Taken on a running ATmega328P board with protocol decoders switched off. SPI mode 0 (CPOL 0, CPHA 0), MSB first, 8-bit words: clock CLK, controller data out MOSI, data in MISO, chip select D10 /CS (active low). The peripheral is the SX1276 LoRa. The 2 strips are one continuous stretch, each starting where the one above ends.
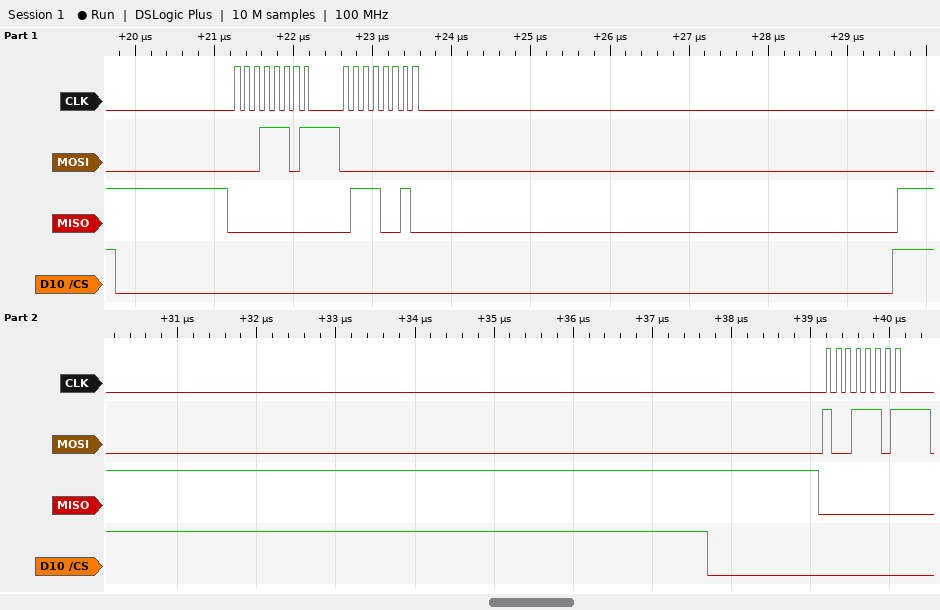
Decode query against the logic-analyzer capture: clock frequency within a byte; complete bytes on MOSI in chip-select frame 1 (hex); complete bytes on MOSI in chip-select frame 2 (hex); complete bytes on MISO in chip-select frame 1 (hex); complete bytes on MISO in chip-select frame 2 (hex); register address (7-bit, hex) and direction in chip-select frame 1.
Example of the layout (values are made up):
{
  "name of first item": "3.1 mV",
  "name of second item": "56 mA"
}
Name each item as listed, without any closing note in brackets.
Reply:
{
  "clock frequency within a byte": "8 MHz",
  "complete bytes on MOSI in chip-select frame 1": "0x1D 0x00",
  "complete bytes on MOSI in chip-select frame 2": "0x9D",
  "complete bytes on MISO in chip-select frame 1": "0x00 0x72",
  "complete bytes on MISO in chip-select frame 2": "0x00",
  "register address (7-bit, hex) and direction in chip-select frame 1": "0x1D read"
}
